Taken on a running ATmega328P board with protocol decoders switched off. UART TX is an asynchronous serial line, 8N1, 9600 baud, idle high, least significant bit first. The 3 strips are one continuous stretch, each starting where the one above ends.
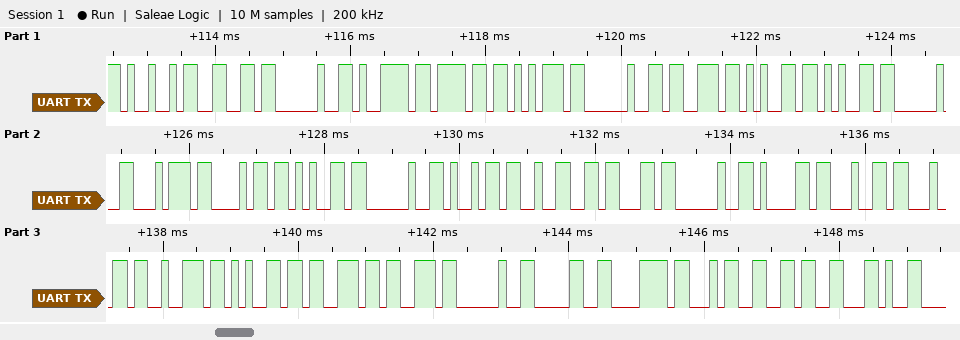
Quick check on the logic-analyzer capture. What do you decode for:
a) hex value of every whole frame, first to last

0x49 0x66 0x20 0x79 0x6F 0x75 0x20 0x73 0x65 0x65 0x20 0x74 0x68 0x65 0x20 0x69 0x32 0x63 0x20 0x61 0x64 0x64 0x72 0x65 0x73 0x73 0x20 0x30 0x78 0x34 0x36 0x2C
